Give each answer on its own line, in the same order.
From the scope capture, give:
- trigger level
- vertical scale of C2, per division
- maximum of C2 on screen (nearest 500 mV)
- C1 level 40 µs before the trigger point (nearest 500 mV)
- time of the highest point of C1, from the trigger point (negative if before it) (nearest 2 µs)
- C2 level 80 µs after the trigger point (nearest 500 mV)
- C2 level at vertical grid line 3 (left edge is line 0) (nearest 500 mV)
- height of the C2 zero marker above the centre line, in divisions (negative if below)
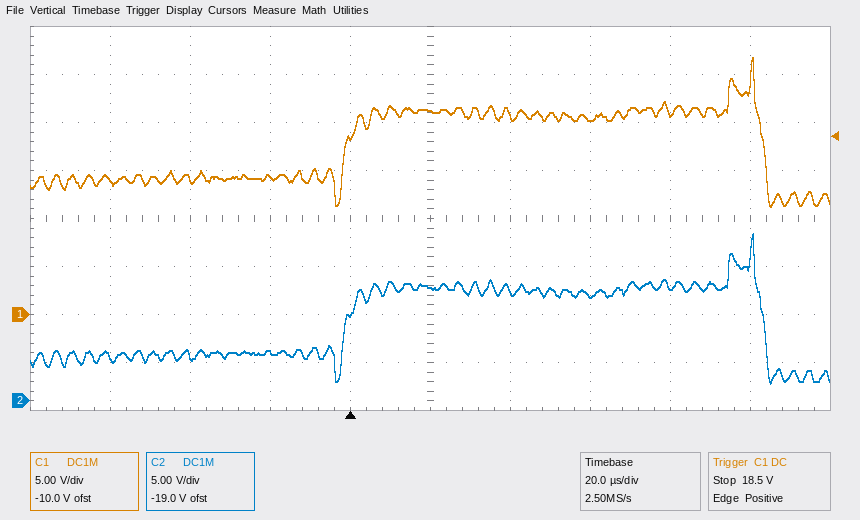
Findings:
18.5 V
5 V
17.5 V
14.0 V
+100 µs
12.0 V
5.0 V
-3.8 div
